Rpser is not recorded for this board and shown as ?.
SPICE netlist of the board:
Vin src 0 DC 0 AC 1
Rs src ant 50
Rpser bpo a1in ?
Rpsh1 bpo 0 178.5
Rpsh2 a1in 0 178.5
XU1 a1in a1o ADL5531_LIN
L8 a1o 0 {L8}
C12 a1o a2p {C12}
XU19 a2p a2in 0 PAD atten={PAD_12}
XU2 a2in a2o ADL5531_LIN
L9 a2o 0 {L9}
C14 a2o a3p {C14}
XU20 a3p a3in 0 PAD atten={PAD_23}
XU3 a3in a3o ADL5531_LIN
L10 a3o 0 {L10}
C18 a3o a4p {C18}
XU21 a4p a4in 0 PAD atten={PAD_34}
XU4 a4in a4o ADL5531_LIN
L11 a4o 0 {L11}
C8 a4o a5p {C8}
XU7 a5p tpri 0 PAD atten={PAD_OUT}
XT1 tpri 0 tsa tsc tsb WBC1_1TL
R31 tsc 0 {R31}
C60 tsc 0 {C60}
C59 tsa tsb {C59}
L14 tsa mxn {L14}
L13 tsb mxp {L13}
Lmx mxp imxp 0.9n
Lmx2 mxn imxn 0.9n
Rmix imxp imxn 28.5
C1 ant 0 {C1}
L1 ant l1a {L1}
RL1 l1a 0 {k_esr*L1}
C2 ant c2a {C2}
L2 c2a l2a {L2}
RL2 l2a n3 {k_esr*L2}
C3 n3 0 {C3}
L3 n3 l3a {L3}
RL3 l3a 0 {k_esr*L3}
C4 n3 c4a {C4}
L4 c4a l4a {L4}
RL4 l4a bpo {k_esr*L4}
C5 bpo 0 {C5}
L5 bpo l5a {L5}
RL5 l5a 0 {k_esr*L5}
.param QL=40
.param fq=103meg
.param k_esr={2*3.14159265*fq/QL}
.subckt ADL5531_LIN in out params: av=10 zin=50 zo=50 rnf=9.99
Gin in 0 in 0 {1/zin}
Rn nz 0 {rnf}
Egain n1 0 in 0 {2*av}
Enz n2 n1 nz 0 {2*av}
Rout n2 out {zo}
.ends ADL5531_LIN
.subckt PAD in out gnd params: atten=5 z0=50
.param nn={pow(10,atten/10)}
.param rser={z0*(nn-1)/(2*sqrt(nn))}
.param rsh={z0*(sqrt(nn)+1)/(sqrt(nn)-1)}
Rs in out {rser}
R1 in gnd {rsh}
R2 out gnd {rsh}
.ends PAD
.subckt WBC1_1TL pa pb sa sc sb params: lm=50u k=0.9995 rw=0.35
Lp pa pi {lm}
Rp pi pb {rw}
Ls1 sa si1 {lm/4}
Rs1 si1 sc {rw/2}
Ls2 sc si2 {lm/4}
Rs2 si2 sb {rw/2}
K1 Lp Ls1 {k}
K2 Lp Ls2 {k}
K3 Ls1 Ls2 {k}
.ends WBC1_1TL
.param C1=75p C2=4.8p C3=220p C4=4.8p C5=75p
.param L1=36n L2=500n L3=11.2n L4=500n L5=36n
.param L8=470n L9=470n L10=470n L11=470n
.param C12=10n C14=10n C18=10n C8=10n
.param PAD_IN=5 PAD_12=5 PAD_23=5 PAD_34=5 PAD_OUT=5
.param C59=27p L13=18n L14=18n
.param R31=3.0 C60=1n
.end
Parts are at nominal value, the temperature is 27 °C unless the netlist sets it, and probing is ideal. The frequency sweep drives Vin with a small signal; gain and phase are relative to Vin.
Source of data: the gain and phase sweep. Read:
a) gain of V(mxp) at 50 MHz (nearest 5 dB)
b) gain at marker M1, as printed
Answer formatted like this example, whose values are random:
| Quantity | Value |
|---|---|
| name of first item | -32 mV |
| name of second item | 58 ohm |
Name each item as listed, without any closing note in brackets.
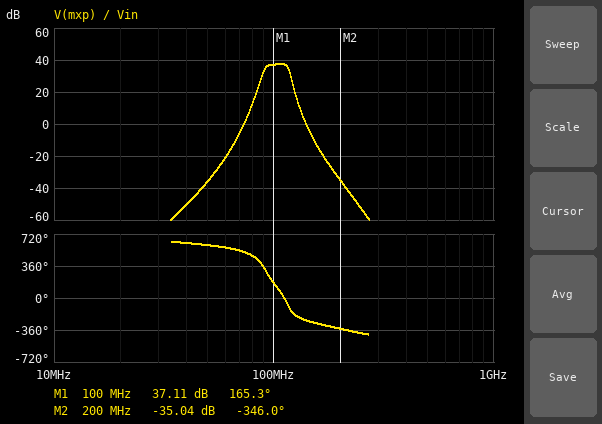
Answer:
| Quantity | Value |
|---|---|
| gain of V(mxp) at 50 MHz | -35 dB |
| gain at marker M1, as printed | 37.11 dB |
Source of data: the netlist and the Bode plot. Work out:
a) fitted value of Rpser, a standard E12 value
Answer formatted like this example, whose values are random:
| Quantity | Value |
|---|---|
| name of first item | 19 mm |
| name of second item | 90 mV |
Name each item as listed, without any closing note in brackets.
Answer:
| Quantity | Value |
|---|---|
| fitted value of Rpser, a standard E12 value | 27 Ω |
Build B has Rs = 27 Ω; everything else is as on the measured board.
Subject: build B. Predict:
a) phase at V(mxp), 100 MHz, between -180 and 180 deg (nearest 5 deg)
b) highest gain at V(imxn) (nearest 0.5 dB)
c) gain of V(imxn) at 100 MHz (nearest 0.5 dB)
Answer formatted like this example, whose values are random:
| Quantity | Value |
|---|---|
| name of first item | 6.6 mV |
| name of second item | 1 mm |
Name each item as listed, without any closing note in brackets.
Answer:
| Quantity | Value |
|---|---|
| phase at V(mxp), 100 MHz, between -180 and 180 deg | 170 deg |
| highest gain at V(imxn) | 40.0 dB |
| gain of V(imxn) at 100 MHz | 39.0 dB |
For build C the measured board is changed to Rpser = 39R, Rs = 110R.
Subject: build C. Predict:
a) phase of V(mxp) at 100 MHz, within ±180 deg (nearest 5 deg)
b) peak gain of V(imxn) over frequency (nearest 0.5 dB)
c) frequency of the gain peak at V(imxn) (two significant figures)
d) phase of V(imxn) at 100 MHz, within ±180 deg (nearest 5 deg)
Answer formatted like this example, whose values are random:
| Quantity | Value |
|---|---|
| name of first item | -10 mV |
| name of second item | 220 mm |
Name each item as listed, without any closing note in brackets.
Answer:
| Quantity | Value |
|---|---|
| phase of V(mxp) at 100 MHz, within ±180 deg | 160 deg |
| peak gain of V(imxn) over frequency | 32.5 dB |
| frequency of the gain peak at V(imxn) | 98 MHz |
| phase of V(imxn) at 100 MHz, within ±180 deg | -25 deg |
